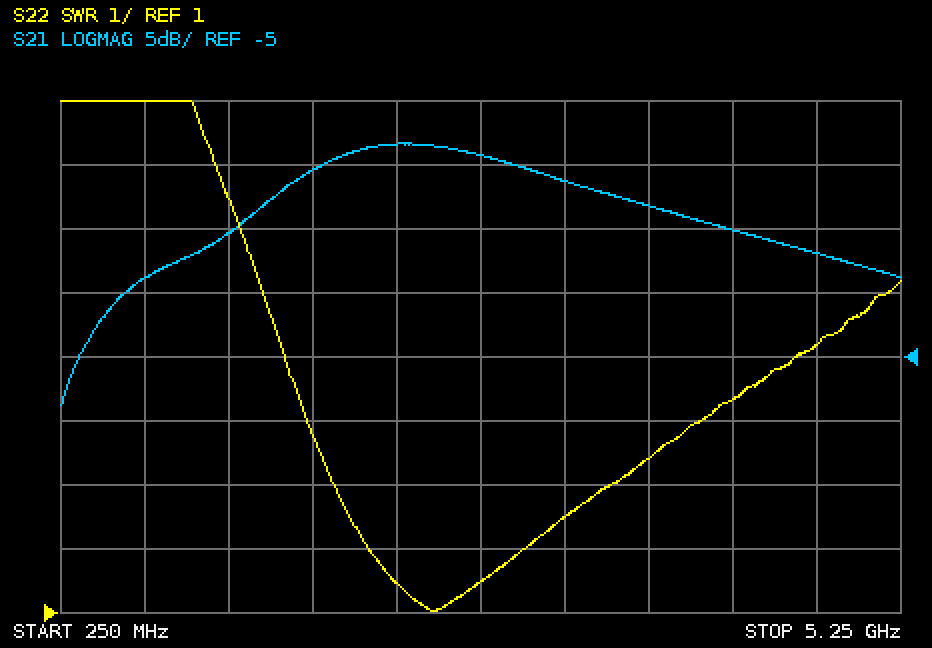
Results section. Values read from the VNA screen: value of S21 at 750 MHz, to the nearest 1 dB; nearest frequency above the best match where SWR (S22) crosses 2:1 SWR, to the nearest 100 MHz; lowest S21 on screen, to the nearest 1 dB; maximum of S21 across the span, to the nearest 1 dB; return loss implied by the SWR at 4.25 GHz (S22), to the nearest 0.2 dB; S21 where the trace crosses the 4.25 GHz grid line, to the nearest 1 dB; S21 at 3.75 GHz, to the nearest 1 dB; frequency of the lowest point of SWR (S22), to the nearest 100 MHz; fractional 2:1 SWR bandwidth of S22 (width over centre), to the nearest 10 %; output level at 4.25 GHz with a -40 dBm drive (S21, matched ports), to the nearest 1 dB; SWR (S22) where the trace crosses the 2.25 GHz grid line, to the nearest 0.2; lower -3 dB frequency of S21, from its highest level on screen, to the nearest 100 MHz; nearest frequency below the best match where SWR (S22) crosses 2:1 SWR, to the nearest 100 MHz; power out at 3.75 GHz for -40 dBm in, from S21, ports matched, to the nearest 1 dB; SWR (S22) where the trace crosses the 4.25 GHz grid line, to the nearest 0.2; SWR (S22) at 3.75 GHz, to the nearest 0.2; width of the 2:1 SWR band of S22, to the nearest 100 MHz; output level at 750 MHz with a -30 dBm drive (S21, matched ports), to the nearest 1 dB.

1 dB
3.0 GHz
-9 dB
12 dB
4.0 dB
5 dB
7 dB
2.5 GHz
40 %
-35 dBm
1.4
1.6 GHz
2.1 GHz
-33 dBm
4.4
3.4
900 MHz
-29 dBm
